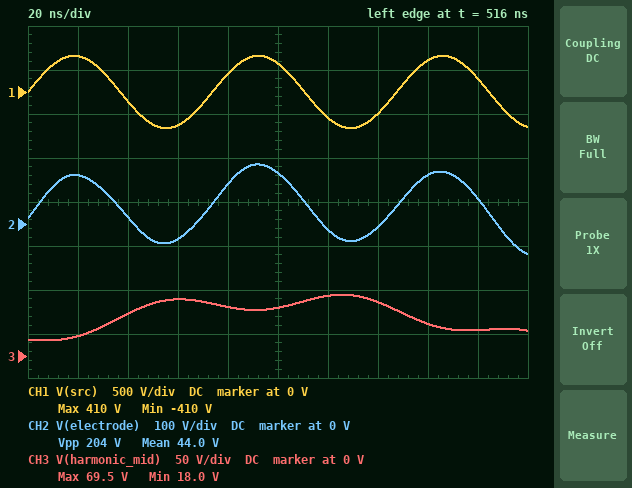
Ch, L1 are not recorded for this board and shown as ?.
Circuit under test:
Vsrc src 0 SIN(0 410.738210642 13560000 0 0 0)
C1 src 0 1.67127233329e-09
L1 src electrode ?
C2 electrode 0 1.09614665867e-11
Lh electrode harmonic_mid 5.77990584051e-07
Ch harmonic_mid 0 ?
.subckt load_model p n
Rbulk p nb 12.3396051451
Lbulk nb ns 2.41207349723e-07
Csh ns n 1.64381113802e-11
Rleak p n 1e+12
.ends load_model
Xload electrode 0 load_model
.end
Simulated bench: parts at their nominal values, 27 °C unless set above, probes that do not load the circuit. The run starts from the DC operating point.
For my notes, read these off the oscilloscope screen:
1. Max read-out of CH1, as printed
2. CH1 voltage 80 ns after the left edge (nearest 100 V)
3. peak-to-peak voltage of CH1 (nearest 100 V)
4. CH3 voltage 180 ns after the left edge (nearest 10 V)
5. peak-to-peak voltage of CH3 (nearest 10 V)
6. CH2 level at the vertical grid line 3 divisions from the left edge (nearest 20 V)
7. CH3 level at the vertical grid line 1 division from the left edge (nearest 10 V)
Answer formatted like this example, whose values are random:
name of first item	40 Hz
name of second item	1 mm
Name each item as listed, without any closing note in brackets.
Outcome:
Max read-out of CH1, as printed	410 V
CH1 voltage 80 ns after the left edge	200 V
peak-to-peak voltage of CH1	800 V
CH3 voltage 180 ns after the left edge	30 V
peak-to-peak voltage of CH3	50 V
CH2 level at the vertical grid line 3 divisions from the left edge	-40 V
CH3 level at the vertical grid line 1 division from the left edge	20 V
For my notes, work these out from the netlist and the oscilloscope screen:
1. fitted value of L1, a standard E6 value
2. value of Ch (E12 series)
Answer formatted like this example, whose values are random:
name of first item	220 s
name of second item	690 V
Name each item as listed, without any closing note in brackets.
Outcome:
fitted value of L1, a standard E6 value	2.2 µH
value of Ch	2.2 nF
